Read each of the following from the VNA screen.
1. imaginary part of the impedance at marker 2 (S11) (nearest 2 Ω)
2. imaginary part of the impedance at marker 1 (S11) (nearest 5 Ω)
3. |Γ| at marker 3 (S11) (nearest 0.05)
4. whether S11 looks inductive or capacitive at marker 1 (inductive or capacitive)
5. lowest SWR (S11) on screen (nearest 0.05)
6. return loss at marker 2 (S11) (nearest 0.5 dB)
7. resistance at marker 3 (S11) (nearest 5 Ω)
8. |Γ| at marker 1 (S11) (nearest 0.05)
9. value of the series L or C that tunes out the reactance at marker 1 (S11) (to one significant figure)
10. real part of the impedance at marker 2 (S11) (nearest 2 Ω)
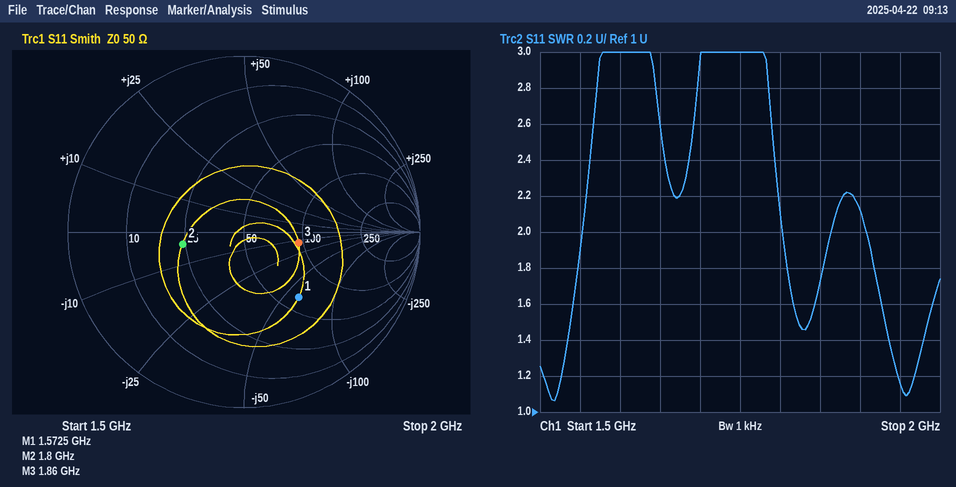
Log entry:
-4 Ω
-60 Ω
0.30
capacitive
1.05
9.0 dB
95 Ω
0.50
6 nH
24 Ω
